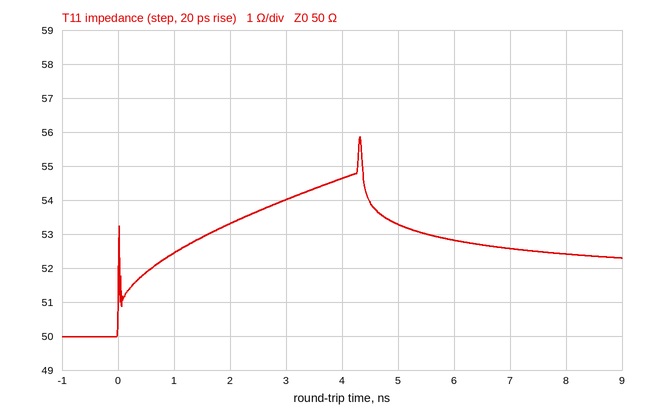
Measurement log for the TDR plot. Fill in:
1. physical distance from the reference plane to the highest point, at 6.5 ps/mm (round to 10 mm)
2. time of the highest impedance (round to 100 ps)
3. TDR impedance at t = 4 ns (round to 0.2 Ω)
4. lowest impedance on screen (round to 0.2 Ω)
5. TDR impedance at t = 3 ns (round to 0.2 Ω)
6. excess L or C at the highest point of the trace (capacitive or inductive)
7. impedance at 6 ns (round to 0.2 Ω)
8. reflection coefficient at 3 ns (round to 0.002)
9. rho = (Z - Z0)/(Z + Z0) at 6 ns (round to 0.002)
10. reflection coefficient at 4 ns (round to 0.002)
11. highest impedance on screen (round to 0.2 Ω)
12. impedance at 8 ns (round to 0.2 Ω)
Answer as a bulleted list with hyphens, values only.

- 330 mm
- 4.3 ns
- 54.6 Ω
- 50.0 Ω
- 54.0 Ω
- inductive
- 52.8 Ω
- +0.038
- +0.028
- +0.044
- 55.8 Ω
- 52.4 Ω
